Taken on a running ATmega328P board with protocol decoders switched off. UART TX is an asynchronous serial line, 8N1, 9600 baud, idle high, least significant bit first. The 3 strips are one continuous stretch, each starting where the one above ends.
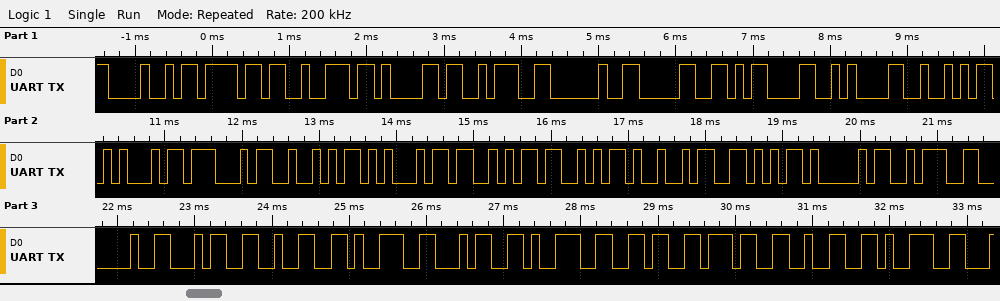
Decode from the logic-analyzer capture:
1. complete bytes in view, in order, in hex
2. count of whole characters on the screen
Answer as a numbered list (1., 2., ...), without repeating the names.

1. 48 6F 72 61 3A 20 30 0D 0A 52 45 47 52 45 53 53 49 56 41 3A 20 34 32 39 34 39 36 37 32 39
2. 30
